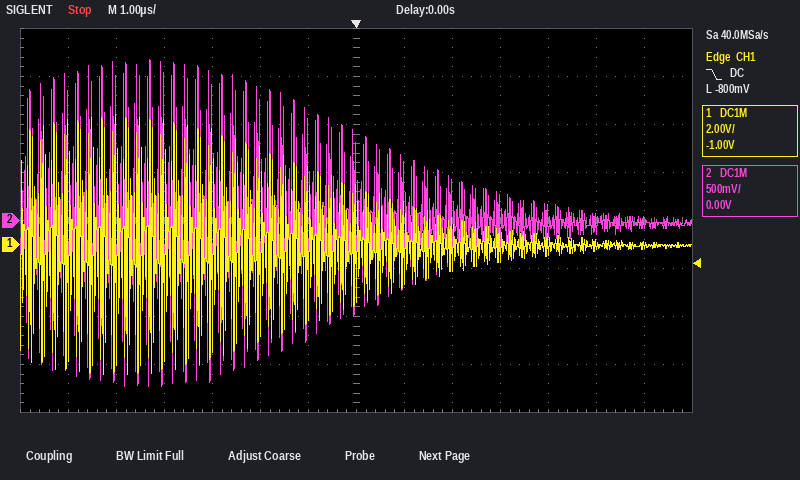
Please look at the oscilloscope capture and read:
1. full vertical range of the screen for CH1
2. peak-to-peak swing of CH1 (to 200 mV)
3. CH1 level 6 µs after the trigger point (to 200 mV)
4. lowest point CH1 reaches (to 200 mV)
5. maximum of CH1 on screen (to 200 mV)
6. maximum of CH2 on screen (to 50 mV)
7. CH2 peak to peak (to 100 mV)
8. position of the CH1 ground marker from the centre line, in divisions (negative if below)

16 V
10.8 V
0.0 V
-5.4 V
5.4 V
1.70 V
3.40 V
-0.5 div
